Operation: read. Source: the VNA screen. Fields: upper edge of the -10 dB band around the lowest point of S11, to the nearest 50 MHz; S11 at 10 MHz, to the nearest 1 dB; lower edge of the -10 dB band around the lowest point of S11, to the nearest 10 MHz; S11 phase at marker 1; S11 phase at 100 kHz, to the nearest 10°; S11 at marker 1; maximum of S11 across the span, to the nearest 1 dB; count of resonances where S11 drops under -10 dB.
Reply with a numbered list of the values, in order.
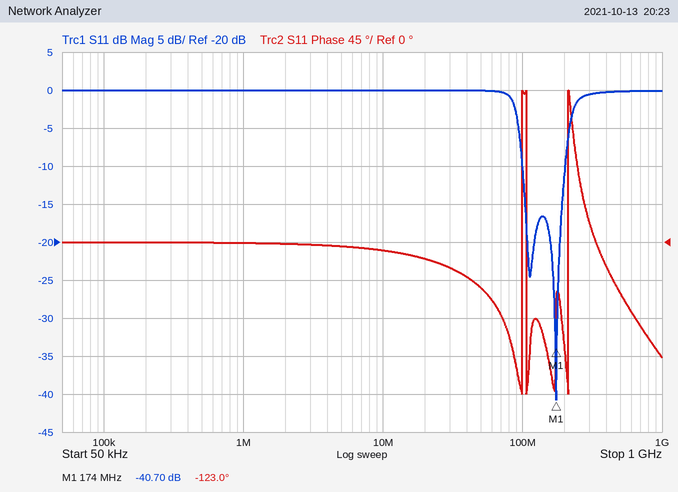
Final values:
1. 200 MHz
2. 0 dB
3. 100 MHz
4. -123.0°
5. 0°
6. -40.70 dB
7. 0 dB
8. 2
